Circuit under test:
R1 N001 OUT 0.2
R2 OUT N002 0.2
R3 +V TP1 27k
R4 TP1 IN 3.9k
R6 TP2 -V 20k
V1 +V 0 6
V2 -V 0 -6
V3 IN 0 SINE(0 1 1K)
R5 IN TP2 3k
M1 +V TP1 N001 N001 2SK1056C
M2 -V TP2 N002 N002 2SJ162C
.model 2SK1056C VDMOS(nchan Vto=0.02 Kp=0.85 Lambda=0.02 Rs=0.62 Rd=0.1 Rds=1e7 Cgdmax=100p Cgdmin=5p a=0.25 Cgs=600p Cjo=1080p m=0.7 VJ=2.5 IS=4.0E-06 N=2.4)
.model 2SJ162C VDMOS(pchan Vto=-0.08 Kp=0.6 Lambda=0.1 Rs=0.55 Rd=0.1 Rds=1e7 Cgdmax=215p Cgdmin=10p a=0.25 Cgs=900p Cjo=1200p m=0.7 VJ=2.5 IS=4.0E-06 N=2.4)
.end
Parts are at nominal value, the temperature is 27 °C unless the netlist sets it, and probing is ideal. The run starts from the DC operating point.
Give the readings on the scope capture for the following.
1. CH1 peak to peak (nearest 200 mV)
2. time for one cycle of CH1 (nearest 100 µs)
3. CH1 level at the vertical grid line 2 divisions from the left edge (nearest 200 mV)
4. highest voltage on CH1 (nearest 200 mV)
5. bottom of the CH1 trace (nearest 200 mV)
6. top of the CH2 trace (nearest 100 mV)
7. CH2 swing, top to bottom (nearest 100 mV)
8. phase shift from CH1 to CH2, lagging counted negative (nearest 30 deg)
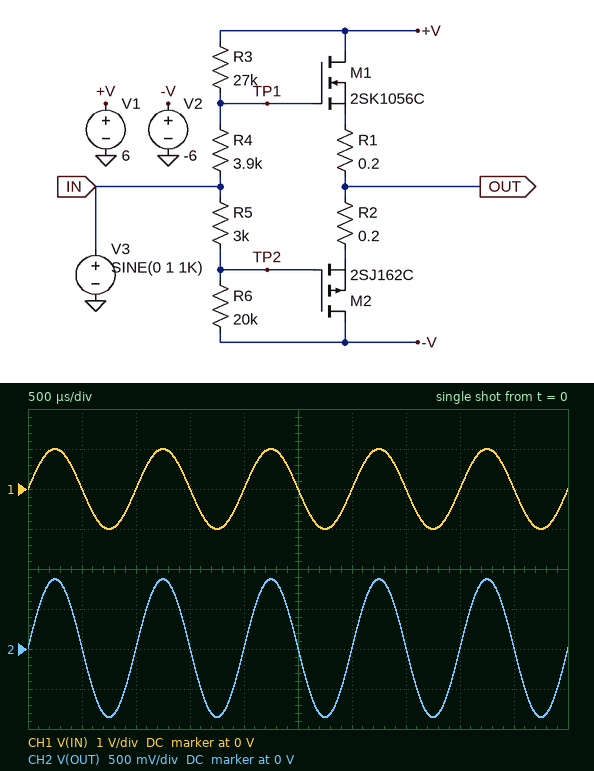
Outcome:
2.0 V
1.0 ms
0 V
1.0 V
-1.0 V
900 mV
1.7 V
0 deg
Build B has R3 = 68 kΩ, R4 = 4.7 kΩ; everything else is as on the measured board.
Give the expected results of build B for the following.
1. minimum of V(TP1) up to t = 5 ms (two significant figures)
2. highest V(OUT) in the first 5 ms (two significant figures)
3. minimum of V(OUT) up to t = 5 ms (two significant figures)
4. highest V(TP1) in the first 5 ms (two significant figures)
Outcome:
-550 mV
720 mV
-1.1 V
1.3 V
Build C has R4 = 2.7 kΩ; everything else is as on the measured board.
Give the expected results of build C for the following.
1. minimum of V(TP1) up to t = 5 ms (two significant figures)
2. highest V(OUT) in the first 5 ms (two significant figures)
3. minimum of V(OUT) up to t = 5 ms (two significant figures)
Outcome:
-360 mV
790 mV
-970 mV
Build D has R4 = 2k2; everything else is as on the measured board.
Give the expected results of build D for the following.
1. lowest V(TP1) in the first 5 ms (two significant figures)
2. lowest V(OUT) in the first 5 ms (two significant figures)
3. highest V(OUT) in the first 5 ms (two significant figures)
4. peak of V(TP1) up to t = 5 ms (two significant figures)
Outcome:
-470 mV
-1.0 V
750 mV
1.4 V
